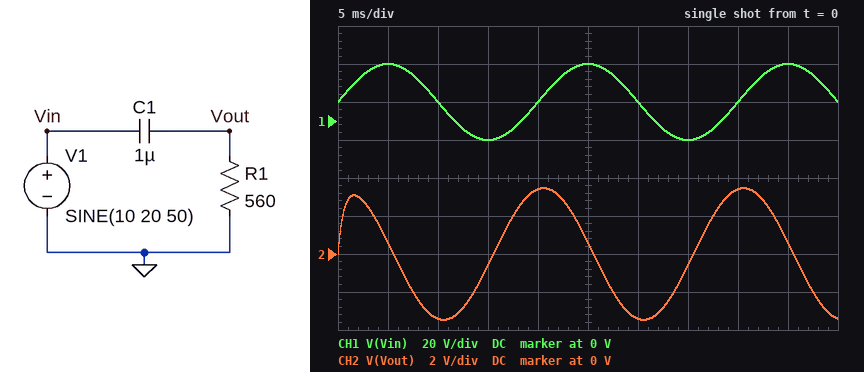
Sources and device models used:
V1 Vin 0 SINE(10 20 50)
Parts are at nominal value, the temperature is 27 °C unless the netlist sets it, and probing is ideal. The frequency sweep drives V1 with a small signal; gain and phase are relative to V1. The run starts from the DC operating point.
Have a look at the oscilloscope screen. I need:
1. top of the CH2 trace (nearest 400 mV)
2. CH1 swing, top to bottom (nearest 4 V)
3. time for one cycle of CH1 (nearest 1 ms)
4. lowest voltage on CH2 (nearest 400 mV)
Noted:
3.6 V
40 V
20 ms
-3.6 V
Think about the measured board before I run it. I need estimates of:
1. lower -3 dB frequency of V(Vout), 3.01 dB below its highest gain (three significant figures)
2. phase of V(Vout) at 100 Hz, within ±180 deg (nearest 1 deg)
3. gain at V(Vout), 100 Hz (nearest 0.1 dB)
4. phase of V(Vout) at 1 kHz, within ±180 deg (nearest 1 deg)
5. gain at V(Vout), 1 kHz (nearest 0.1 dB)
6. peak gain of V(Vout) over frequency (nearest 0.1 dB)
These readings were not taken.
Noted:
284 Hz
71 deg
-9.6 dB
16 deg
-0.3 dB
0 dB
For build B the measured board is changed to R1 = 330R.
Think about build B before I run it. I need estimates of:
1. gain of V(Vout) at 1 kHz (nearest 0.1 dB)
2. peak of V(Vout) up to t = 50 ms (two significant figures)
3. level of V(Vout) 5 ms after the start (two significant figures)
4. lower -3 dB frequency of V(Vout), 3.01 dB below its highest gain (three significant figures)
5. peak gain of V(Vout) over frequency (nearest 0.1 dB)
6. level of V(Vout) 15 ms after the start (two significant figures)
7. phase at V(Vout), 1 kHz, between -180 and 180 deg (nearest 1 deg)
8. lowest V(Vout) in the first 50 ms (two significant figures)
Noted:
-0.9 dB
2.1 V
210 mV
482 Hz
0 dB
-210 mV
26 deg
-2.1 V
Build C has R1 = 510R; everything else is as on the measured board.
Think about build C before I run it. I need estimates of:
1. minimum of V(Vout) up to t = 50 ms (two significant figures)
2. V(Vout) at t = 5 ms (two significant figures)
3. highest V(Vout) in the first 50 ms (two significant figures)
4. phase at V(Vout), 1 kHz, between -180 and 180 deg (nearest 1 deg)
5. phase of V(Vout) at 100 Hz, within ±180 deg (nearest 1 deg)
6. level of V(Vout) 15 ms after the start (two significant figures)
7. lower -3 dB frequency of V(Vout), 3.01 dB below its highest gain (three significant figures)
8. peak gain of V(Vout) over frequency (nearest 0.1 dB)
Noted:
-3.2 V
500 mV
3.2 V
17 deg
72 deg
-500 mV
312 Hz
0 dB
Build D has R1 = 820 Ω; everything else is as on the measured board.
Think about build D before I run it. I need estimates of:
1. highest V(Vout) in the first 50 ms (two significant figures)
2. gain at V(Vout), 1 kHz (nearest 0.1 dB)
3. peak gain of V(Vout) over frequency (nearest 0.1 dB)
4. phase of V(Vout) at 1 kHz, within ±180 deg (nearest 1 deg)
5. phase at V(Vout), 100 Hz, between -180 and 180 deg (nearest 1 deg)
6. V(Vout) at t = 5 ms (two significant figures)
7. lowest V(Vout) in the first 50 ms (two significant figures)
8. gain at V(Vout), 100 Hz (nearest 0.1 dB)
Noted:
5.0 V
-0.2 dB
0 dB
11 deg
63 deg
1.2 V
-5.0 V
-6.8 dB
